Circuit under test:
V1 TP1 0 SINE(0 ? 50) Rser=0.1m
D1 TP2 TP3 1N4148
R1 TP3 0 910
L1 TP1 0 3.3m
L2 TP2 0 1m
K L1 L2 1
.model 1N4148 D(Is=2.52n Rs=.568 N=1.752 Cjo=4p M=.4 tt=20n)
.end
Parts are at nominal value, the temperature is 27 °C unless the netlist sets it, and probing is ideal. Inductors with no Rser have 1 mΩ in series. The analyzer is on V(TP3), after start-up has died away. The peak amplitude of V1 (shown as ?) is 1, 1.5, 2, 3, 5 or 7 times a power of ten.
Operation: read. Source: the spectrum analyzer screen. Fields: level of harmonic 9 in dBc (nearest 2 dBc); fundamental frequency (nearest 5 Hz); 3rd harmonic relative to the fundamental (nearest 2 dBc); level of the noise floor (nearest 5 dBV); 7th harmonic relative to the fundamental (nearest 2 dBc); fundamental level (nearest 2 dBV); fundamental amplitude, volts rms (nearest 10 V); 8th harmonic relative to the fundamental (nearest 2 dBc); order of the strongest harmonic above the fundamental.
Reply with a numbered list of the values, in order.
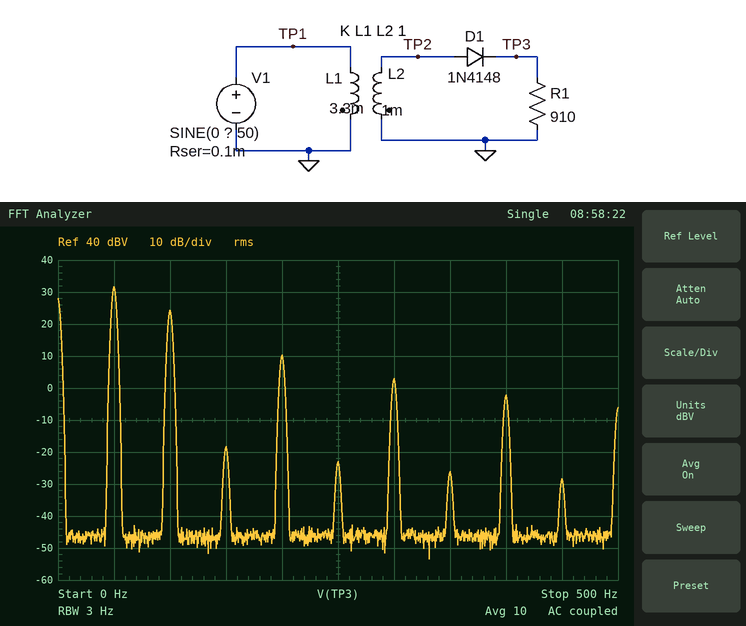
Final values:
1. -60 dBc
2. 50 Hz
3. -50 dBc
4. -45 dBV
5. -58 dBc
6. 32 dBV
7. 40 V
8. -34 dBc
9. 2
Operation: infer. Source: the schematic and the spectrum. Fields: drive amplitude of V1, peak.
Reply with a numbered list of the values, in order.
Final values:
1. 200 V
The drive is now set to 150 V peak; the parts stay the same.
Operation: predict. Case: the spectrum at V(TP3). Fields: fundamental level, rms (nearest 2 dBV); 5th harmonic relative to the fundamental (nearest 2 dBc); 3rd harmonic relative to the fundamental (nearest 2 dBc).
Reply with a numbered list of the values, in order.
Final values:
1. 30 dBV
2. -52 dBc
3. -48 dBc
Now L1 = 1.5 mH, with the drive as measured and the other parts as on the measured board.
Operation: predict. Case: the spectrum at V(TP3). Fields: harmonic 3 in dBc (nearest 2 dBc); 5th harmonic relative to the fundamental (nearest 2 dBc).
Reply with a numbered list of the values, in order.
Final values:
1. -52 dBc
2. -56 dBc
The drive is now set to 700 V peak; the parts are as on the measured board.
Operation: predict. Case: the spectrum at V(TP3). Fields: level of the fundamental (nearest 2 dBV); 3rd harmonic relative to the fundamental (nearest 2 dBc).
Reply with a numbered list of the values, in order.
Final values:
1. 42 dBV
2. -58 dBc
